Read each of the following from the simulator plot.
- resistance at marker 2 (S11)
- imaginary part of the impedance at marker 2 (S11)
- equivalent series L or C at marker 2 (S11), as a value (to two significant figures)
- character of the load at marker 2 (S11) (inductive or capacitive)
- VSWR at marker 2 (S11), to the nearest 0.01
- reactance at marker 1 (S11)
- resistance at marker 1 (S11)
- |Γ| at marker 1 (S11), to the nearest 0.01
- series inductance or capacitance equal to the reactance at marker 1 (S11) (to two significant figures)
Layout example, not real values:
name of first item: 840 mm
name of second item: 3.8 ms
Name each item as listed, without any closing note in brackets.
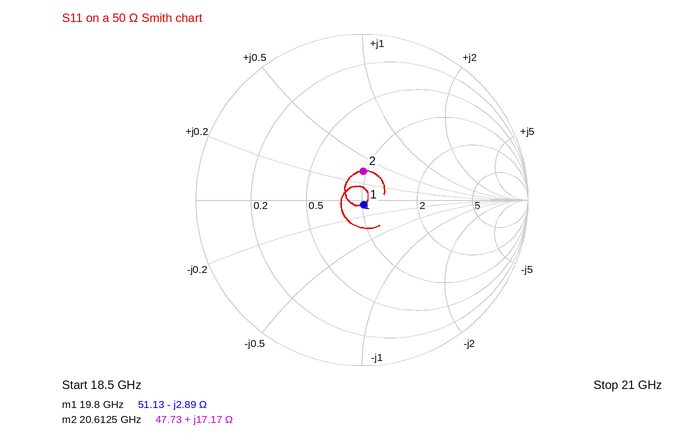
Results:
resistance at marker 2: 47.73 Ω
imaginary part of the impedance at marker 2: +17.17 Ω
equivalent series L or C at marker 2 (S11), as a value: 130 pH
character of the load at marker 2 (S11): inductive
VSWR at marker 2 (S11), to the nearest 0.01: 1.42
reactance at marker 1: -2.89 Ω
resistance at marker 1: 51.13 Ω
|Γ| at marker 1 (S11), to the nearest 0.01: 0.03
series inductance or capacitance equal to the reactance at marker 1 (S11): 2.8 pF
